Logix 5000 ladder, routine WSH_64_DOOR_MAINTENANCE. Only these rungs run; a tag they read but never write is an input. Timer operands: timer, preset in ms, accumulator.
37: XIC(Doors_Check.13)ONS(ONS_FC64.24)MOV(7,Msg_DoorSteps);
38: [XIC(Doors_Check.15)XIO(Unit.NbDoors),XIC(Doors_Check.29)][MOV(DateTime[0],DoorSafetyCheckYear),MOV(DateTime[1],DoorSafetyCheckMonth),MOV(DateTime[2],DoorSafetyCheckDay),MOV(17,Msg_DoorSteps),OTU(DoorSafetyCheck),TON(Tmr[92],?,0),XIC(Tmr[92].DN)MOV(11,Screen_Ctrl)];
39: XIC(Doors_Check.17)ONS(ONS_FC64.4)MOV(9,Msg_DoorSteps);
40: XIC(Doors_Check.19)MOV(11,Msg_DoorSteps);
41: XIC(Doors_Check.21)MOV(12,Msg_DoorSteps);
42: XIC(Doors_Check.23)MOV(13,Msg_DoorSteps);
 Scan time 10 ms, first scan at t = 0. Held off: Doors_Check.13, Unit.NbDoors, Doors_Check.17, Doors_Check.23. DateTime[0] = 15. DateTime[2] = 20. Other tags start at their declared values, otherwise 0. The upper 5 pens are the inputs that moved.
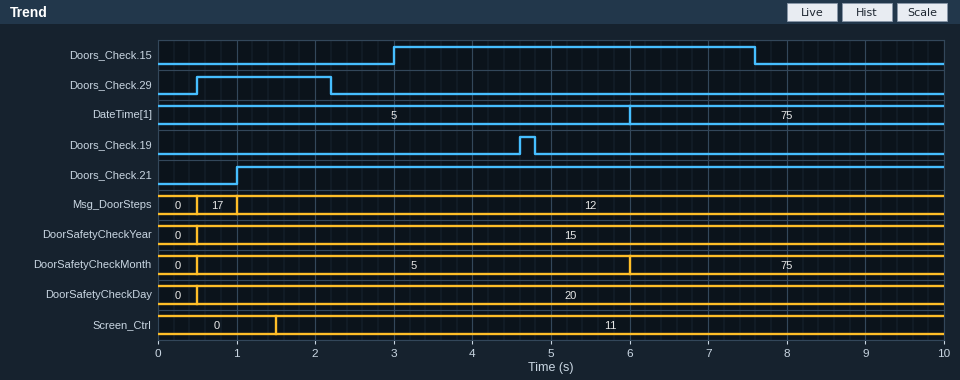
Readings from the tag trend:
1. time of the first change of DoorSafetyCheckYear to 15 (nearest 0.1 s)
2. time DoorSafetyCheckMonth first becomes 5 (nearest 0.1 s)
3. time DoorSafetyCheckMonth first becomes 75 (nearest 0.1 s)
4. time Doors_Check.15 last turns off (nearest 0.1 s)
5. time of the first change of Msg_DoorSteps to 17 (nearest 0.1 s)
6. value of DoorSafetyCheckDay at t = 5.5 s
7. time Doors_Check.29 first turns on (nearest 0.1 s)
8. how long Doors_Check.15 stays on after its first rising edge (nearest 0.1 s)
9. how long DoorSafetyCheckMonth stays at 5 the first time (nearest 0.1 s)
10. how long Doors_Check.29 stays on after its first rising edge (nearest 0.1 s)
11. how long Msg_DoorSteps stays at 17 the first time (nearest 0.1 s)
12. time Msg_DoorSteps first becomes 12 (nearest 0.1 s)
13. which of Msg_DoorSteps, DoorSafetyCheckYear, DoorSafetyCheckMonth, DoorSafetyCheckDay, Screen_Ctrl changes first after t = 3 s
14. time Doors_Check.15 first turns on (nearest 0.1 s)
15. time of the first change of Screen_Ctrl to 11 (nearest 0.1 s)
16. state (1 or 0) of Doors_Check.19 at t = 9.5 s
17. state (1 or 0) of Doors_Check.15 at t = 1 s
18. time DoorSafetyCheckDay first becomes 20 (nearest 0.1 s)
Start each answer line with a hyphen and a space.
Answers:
- 0.5 s
- 0.5 s
- 6.0 s
- 7.6 s
- 0.5 s
- 20
- 0.5 s
- 4.6 s
- 5.5 s
- 1.7 s
- 0.5 s
- 1.0 s
- DoorSafetyCheckMonth
- 3.0 s
- 1.5 s
- 0
- 0
- 0.5 s
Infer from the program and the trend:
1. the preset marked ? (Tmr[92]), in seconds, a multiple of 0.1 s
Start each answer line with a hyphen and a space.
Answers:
- 1.0 s
